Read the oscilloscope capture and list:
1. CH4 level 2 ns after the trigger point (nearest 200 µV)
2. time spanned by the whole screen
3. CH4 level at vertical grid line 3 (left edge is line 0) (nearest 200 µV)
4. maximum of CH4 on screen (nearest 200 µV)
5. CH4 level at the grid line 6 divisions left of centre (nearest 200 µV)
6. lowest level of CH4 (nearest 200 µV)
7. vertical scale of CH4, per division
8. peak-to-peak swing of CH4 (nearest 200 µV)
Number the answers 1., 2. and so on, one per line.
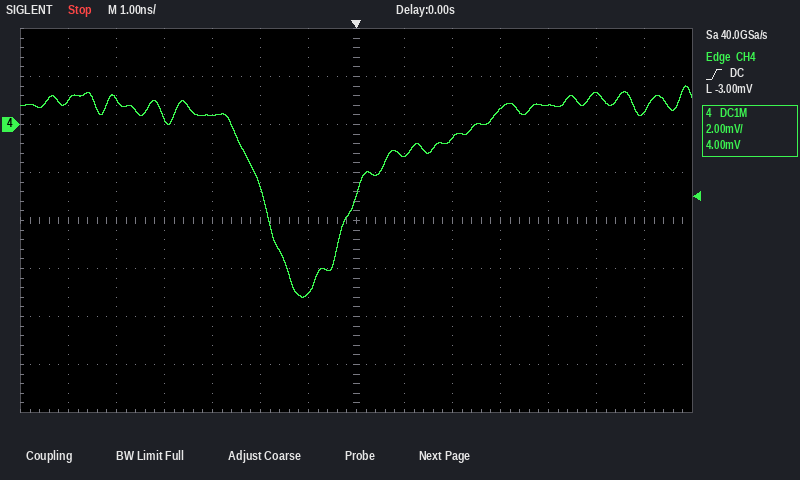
1. -600 µV
2. 14 ns
3. 200 µV
4. 1.6 mV
5. 1.0 mV
6. -7.2 mV
7. 2 mV
8. 8.8 mV
